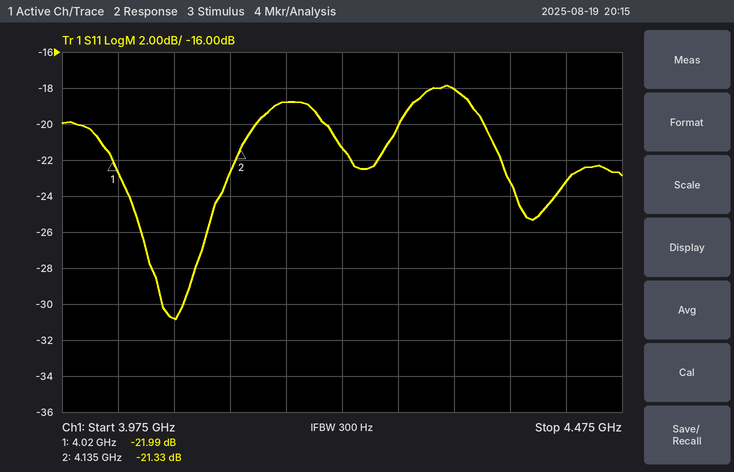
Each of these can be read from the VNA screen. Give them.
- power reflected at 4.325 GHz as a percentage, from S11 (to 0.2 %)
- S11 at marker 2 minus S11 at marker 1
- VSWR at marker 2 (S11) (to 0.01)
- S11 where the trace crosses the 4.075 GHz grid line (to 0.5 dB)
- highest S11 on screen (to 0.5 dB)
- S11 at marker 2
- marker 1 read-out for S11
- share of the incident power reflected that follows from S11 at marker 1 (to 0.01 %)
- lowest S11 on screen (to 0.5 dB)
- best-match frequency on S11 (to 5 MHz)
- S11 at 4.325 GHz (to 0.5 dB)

1.6 %
0.66 dB
1.19
-31.0 dB
-18.0 dB
-21.33 dB
-21.99 dB
0.63 %
-31.0 dB
4.075 GHz
-18.0 dB
